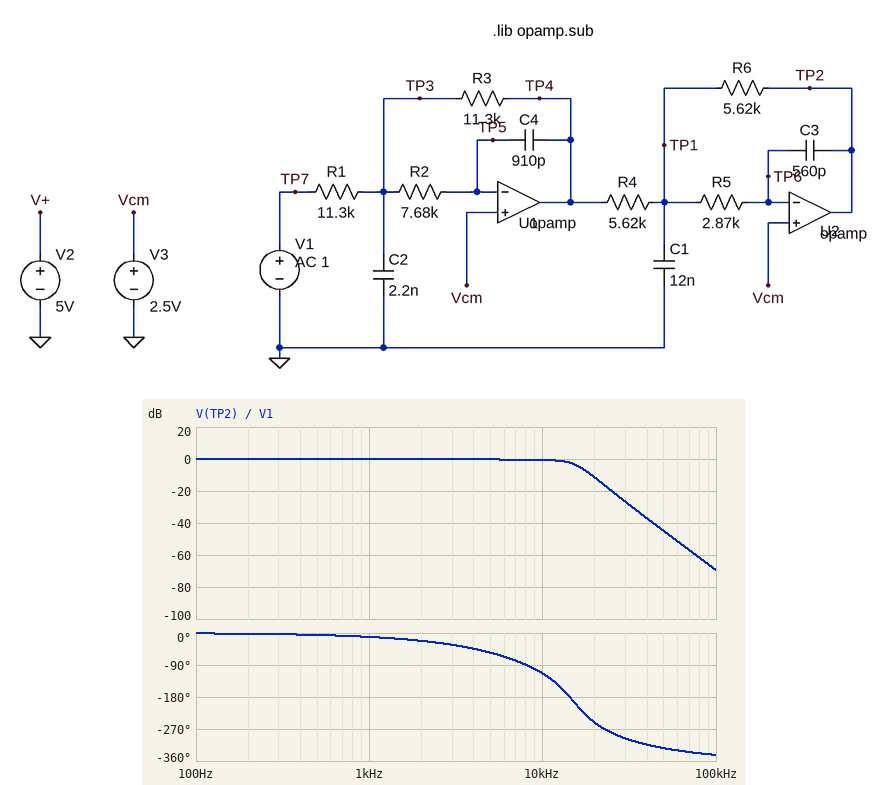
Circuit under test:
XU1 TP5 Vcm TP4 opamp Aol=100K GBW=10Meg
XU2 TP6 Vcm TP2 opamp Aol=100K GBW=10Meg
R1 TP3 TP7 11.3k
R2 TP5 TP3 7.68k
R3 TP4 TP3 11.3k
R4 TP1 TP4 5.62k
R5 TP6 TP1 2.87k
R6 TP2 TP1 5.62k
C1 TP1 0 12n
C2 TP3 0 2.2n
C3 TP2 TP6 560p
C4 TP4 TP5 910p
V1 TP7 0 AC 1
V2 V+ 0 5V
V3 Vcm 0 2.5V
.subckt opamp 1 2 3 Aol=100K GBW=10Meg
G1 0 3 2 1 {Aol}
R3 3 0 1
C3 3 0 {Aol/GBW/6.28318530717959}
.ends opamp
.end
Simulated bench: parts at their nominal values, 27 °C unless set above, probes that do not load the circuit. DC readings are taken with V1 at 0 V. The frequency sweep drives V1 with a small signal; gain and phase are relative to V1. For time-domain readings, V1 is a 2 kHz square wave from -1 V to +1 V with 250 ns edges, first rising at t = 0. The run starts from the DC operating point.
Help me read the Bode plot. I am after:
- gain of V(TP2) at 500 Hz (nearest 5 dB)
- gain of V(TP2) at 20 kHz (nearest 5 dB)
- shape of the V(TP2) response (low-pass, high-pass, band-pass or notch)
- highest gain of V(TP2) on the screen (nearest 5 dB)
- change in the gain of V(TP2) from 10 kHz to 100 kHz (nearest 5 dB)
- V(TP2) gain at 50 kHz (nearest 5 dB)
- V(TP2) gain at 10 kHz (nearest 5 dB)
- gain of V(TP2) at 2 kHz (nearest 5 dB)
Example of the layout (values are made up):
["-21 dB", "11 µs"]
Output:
["0 dB", "-10 dB", "low-pass", "0 dB", "-70 dB", "-45 dB", "0 dB", "0 dB"]
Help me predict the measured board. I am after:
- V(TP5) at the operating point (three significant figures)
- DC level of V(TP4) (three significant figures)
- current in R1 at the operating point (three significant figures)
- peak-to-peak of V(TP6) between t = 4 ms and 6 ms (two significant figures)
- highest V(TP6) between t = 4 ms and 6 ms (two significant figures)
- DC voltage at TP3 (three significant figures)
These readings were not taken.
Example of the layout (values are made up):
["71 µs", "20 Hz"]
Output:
["2.50 V", "5.00 V", "221 µA", "2.2 mV", "2.5 V", "2.50 V"]
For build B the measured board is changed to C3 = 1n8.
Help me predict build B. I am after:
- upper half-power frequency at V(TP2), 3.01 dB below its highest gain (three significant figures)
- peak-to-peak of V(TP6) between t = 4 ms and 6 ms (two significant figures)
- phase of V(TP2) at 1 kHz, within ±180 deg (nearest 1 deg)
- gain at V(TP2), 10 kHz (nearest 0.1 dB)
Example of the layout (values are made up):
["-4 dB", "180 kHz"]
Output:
["8.09 kHz", "1.3 mV", "-16 deg", "-6.4 dB"]
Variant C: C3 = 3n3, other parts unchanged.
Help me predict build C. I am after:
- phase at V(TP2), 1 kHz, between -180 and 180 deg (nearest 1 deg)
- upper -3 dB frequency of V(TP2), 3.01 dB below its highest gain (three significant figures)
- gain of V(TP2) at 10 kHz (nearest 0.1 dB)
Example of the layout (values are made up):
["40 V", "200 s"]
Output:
["-22 deg", "5.10 kHz", "-12.8 dB"]
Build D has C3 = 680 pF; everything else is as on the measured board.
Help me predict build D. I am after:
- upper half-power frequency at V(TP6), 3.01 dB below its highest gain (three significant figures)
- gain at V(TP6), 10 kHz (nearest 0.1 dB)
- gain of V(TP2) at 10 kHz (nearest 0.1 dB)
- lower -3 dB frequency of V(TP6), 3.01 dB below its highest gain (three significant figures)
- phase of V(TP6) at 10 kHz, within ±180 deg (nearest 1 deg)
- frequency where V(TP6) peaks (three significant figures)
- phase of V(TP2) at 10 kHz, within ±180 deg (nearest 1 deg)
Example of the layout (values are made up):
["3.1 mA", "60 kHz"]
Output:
["16.0 kHz", "-60.5 dB", "-0.5 dB", "7.55 kHz", "145 deg", "12.1 kHz", "-124 deg"]
